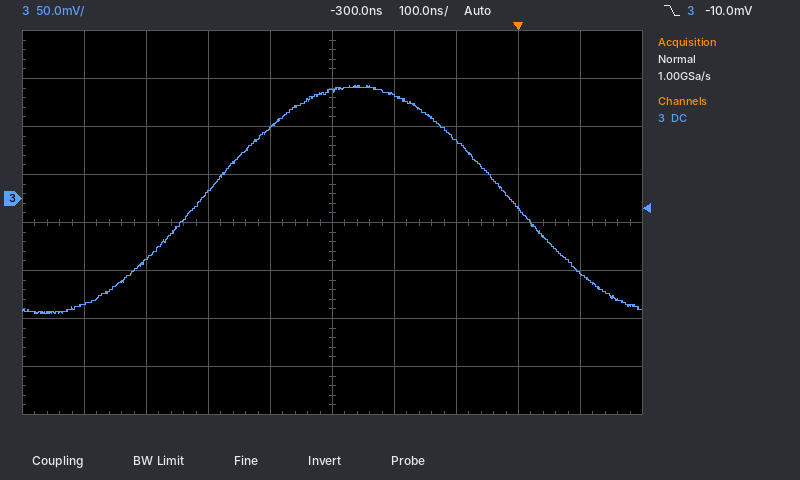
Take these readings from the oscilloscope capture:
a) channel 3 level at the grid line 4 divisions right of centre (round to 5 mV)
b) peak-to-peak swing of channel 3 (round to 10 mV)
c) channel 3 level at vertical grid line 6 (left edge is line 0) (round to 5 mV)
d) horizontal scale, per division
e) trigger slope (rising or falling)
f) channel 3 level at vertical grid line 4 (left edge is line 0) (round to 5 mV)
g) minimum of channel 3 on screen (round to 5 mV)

-80 mV
240 mV
110 mV
100 ns
falling
75 mV
-120 mV
